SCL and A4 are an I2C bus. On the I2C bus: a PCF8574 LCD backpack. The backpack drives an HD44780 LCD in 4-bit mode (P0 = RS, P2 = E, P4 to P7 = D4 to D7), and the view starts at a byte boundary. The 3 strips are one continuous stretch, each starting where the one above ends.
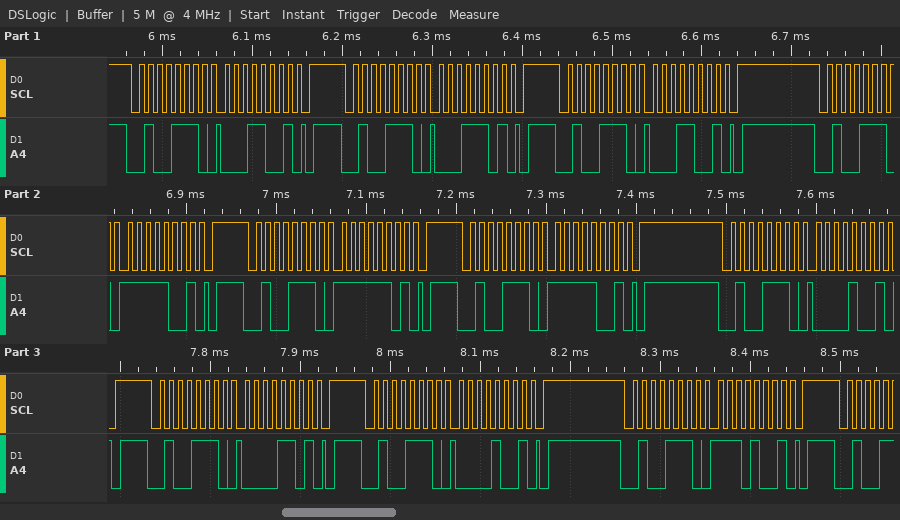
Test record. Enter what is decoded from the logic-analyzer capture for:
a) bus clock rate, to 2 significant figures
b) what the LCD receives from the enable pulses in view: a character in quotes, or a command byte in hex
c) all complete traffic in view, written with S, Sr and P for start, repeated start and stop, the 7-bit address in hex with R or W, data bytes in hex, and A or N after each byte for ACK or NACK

100 kHz
data 0x1F
S 27W A 19 A P S 27W A 1D A P S 27W A 19 A P S 27W A F9 A P S 27W A FD A P S 27W A F9 A P S 27W A 09 A P S 27W A 0D A P S 27W A 09 A P S 27W A E9 A P
